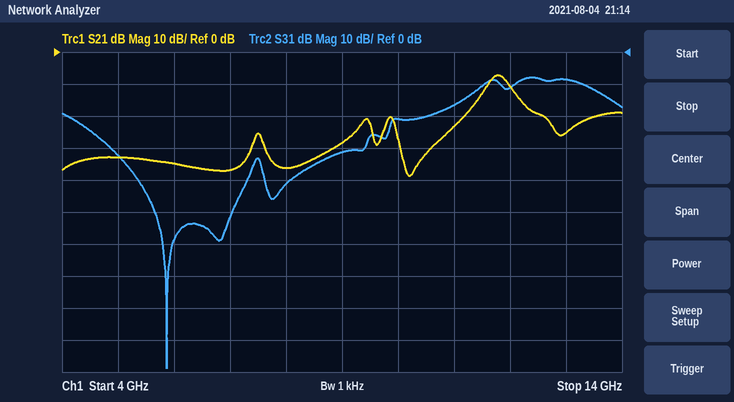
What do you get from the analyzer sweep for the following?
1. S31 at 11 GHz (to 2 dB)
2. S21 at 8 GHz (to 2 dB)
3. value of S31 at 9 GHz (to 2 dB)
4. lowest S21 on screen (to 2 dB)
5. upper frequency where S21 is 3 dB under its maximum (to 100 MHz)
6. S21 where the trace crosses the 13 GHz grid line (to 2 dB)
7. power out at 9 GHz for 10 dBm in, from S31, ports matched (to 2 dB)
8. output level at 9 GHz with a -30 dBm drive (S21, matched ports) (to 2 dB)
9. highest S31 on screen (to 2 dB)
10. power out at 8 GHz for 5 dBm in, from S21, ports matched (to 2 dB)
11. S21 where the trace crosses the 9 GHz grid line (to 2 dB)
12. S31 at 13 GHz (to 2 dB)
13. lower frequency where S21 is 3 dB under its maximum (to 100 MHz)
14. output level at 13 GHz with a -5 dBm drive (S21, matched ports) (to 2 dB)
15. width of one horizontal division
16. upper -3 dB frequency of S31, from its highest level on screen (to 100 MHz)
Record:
-16 dB
-36 dB
-32 dB
-38 dB
12.0 GHz
-26 dB
-22 dBm
-58 dBm
-8 dB
-32 dBm
-28 dB
-8 dB
11.6 GHz
-30 dBm
1 GHz
13.4 GHz
